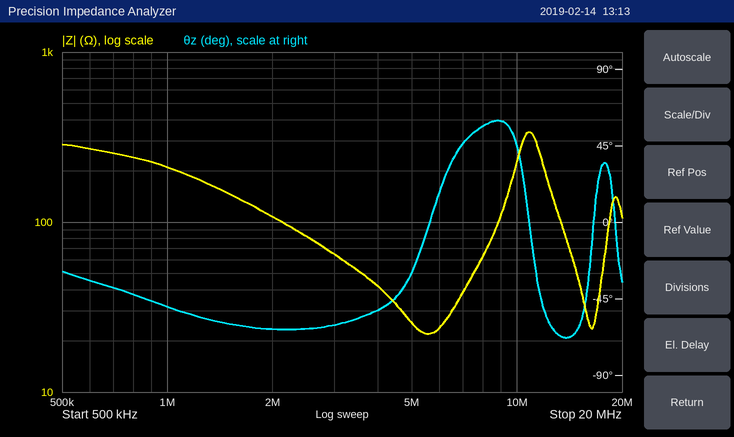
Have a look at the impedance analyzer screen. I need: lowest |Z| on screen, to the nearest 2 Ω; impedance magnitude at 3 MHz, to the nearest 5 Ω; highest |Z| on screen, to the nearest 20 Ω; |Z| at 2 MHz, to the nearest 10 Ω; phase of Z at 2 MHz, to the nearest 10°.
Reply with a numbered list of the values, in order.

1. 22 Ω
2. 65 Ω
3. 340 Ω
4. 110 Ω
5. -60°
